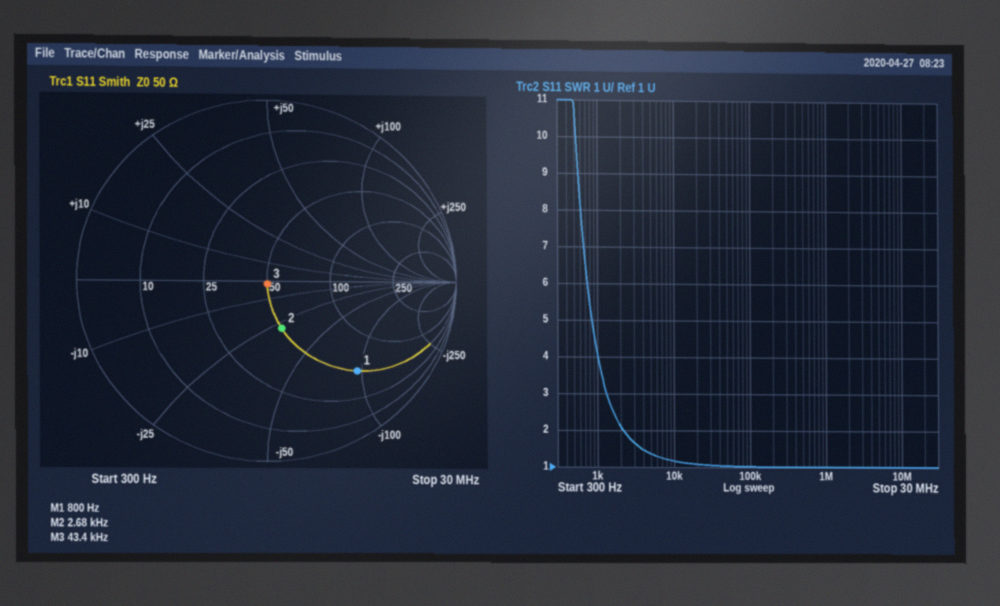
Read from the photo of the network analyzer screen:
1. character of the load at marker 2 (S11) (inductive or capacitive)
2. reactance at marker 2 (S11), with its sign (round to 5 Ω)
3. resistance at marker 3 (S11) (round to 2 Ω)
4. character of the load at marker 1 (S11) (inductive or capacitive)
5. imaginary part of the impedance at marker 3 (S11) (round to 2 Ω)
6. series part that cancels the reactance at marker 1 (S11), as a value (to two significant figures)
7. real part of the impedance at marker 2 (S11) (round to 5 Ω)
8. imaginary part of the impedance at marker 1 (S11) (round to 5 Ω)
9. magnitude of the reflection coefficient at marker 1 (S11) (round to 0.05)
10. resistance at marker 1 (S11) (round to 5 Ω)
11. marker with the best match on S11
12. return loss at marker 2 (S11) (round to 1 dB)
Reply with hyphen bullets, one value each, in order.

- capacitive
- -30 Ω
- 50 Ω
- capacitive
- -2 Ω
- 19 mH
- 50 Ω
- -95 Ω
- 0.70
- 50 Ω
- marker 3
- 11 dB
